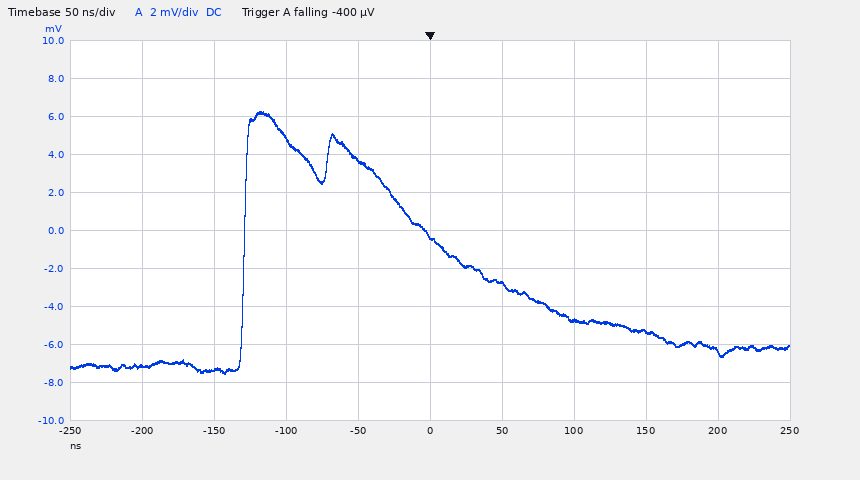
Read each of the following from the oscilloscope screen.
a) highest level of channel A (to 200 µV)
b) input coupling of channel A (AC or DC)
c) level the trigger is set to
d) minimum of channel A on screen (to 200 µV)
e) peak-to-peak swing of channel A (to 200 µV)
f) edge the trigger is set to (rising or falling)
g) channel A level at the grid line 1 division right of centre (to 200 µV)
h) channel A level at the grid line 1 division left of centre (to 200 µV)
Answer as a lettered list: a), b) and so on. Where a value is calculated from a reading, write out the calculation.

a) 6.2 mV
b) DC
c) -400 µV
d) -7.6 mV
e) 6.2 mV − (-7.6 mV) = 13.8 mV
f) falling
g) -2.8 mV
h) 3.8 mV
